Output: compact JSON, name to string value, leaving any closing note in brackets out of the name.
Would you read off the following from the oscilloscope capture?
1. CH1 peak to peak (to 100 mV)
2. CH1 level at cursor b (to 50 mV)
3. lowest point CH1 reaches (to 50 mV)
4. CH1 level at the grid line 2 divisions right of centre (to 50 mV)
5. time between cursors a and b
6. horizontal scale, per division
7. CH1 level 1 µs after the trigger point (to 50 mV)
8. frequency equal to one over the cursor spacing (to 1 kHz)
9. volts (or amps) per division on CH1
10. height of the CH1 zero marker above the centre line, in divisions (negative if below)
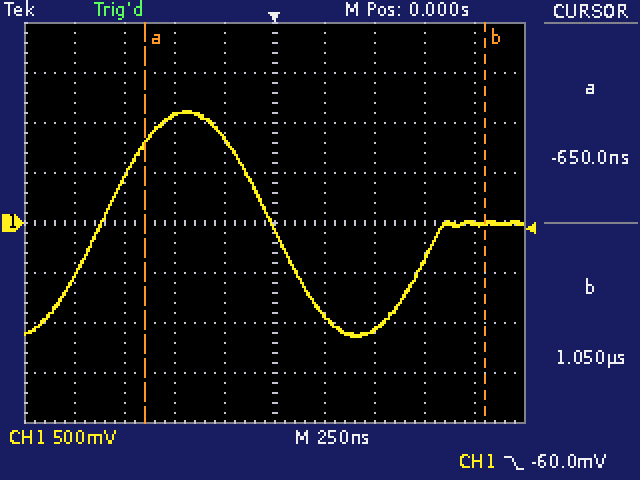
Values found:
{"CH1 peak to peak": "2.30 V", "CH1 level at cursor b": "0 mV", "lowest point CH1 reaches": "-1.15 V", "CH1 level at the grid line 2 divisions right of centre": "-1.05 V", "time between cursors a and b": "1.700 µs", "horizontal scale, per division": "250 ns", "CH1 level 1 µs after the trigger point": "0 mV", "frequency equal to one over the cursor spacing": "588 kHz", "volts (or amps) per division on CH1": "500 mV", "height of the CH1 zero marker above the centre line, in divisions": "0.0 div"}
